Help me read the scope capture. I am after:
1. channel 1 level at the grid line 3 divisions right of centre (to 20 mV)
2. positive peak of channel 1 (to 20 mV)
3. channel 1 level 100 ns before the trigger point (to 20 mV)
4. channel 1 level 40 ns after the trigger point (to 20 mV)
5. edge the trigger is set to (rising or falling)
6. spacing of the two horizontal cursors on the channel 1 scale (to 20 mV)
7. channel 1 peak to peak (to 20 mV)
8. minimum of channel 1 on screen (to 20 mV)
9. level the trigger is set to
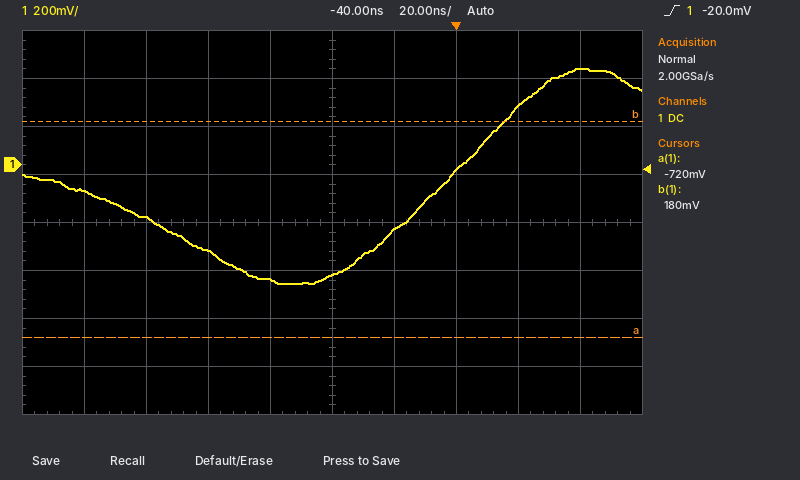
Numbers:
240 mV
400 mV
-220 mV
400 mV
rising
900 mV
900 mV
-500 mV
-20.0 mV
